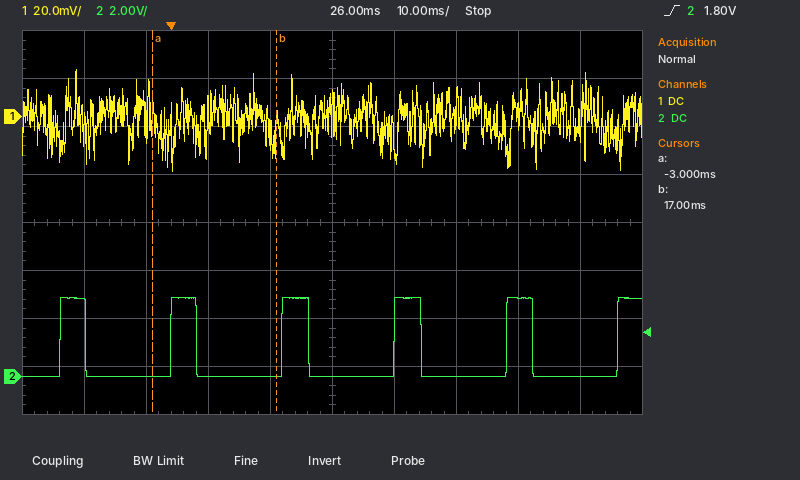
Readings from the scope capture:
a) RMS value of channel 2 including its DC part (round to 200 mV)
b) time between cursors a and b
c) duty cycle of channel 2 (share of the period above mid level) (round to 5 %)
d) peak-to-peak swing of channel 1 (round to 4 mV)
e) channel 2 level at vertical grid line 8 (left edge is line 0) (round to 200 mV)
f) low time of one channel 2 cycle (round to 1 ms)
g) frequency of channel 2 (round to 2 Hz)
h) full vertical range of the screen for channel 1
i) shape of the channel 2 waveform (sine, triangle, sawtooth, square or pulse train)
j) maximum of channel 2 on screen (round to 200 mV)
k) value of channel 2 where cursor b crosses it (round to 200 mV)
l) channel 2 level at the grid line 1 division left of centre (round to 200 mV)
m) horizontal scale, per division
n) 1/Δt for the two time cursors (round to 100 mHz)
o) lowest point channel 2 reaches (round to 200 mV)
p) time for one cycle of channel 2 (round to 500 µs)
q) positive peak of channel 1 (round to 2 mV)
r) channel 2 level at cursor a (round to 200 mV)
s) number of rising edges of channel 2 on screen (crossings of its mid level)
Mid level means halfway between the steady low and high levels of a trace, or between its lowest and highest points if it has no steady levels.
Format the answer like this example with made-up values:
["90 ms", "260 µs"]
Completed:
["1.6 V", "20 ms", "25 %", "44 mV", "3.2 V", "14 ms", "56 Hz", "160 mV", "pulse train", "3.2 V", "0.0 V", "0.0 V", "10 ms", "50.0 Hz", "0.0 V", "18.0 ms", "20 mV", "0.0 V", "6"]
